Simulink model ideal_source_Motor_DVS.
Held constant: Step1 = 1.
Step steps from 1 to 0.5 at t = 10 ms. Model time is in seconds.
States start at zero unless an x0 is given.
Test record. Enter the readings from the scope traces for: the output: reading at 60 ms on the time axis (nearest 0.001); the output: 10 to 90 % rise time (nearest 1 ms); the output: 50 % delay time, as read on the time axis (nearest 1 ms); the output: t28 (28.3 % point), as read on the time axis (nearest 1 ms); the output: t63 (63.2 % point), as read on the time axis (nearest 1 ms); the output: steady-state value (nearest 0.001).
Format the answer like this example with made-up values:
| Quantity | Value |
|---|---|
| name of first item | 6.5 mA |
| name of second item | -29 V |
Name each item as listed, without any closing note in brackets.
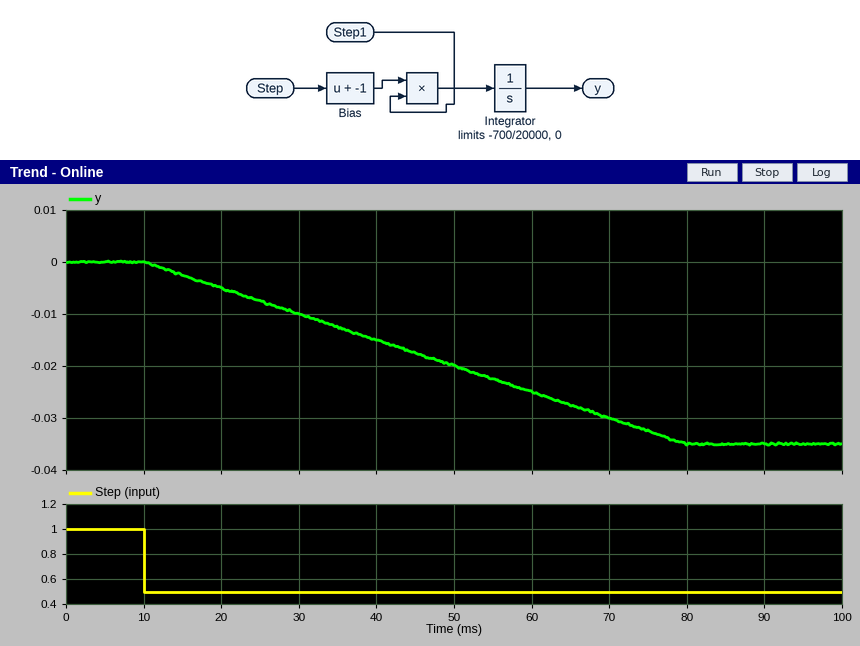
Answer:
| Quantity | Value |
|---|---|
| the output: reading at 60 ms on the time axis | -0.025 |
| the output: 10 to 90 % rise time | 56 ms |
| the output: 50 % delay time, as read on the time axis | 45 ms |
| the output: t28 (28.3 % point), as read on the time axis | 30 ms |
| the output: t63 (63.2 % point), as read on the time axis | 54 ms |
| the output: steady-state value | -0.035 |
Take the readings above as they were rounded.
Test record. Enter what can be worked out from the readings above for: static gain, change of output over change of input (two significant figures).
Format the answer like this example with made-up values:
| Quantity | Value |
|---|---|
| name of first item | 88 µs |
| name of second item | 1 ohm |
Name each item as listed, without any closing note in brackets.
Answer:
| Quantity | Value |
|---|---|
| static gain, change of output over change of input | 0.070 |
